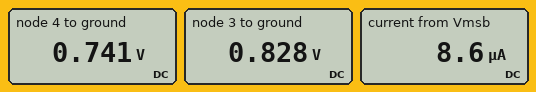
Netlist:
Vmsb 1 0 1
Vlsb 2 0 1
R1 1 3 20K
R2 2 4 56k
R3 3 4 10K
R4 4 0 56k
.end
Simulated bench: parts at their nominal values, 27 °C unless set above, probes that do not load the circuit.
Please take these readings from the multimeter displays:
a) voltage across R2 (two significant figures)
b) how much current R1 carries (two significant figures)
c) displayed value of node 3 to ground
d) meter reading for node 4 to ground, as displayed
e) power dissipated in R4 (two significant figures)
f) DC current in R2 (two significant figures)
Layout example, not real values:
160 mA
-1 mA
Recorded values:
260 mV
8.6 µA
0.828 V
0.741 V
9.8 µW
4.6 µA
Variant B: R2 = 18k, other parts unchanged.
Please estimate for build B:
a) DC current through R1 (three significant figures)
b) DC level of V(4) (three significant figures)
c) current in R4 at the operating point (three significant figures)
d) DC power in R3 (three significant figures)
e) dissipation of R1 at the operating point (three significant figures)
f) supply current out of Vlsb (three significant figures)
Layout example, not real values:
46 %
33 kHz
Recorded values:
5.58 µA
833 mV
14.9 µA
311 nW
622 nW
9.29 µA
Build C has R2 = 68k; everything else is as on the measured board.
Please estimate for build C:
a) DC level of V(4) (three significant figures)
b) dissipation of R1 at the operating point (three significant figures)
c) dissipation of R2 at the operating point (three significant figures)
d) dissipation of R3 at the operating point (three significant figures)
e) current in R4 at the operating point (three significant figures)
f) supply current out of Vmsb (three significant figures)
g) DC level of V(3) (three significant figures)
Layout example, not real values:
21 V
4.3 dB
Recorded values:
729 mV
1.63 µW
1.08 µW
816 nW
13.0 µA
9.03 µA
819 mV
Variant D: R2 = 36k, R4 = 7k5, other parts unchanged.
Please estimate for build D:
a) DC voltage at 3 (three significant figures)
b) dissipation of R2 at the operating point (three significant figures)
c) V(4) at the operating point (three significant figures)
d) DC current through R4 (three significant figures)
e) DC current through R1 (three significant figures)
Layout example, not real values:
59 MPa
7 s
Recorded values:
543 mV
13.1 µW
314 mV
41.9 µA
22.9 µA
